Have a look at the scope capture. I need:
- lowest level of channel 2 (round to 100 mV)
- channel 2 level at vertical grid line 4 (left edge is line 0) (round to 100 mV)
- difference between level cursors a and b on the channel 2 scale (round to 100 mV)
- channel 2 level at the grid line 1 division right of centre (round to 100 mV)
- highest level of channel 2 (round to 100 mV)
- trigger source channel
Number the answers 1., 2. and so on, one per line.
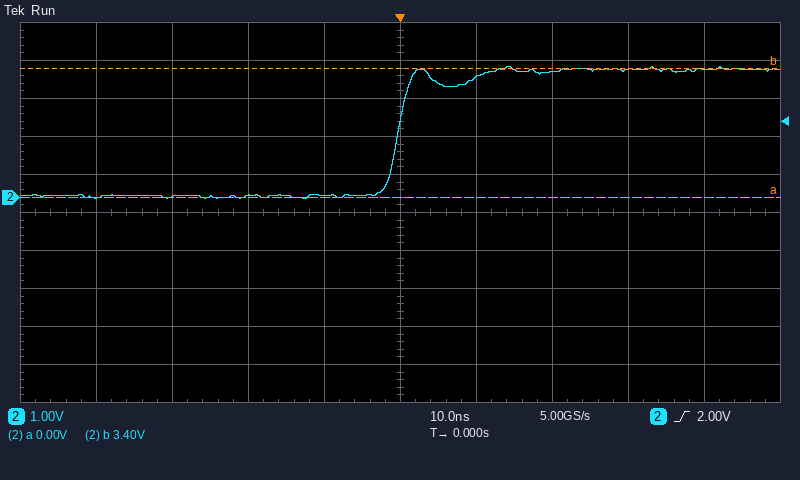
1. 0.0 V
2. 0.0 V
3. 3.4 V
4. 3.1 V
5. 3.4 V
6. channel 2
